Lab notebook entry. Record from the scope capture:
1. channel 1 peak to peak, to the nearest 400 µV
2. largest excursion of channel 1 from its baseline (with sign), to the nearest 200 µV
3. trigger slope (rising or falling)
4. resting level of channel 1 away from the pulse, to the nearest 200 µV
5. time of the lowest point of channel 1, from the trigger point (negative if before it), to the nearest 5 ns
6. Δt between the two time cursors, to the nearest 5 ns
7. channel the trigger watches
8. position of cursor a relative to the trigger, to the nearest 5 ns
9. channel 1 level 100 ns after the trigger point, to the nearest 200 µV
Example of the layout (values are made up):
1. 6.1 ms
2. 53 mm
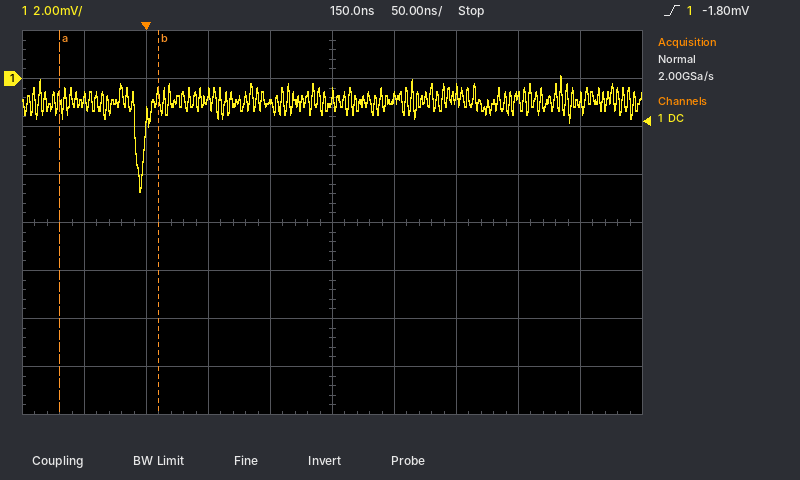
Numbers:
1. 4.8 mV
2. -3.8 mV
3. rising
4. -1.0 mV
5. -5 ns
6. 80 ns
7. channel 1
8. -70 ns
9. -1.0 mV
